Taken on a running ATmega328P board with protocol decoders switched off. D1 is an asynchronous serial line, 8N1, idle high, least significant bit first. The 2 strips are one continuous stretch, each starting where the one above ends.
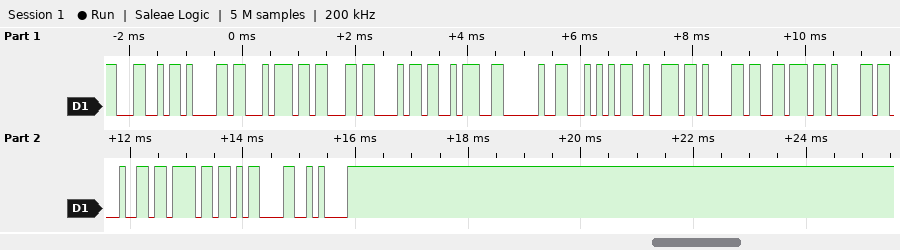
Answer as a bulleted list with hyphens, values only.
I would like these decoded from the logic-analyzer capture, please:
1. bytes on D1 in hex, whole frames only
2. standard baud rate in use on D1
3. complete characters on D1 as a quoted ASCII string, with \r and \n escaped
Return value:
- 0x4C 0x61 0x74 0x63 0x68 0x3A 0x20 0x54 0x72 0x61 0x76 0x61 0x64 0x6F 0x0D 0x0A
- 9600 baud
- "Latch: Travado\r\n"
